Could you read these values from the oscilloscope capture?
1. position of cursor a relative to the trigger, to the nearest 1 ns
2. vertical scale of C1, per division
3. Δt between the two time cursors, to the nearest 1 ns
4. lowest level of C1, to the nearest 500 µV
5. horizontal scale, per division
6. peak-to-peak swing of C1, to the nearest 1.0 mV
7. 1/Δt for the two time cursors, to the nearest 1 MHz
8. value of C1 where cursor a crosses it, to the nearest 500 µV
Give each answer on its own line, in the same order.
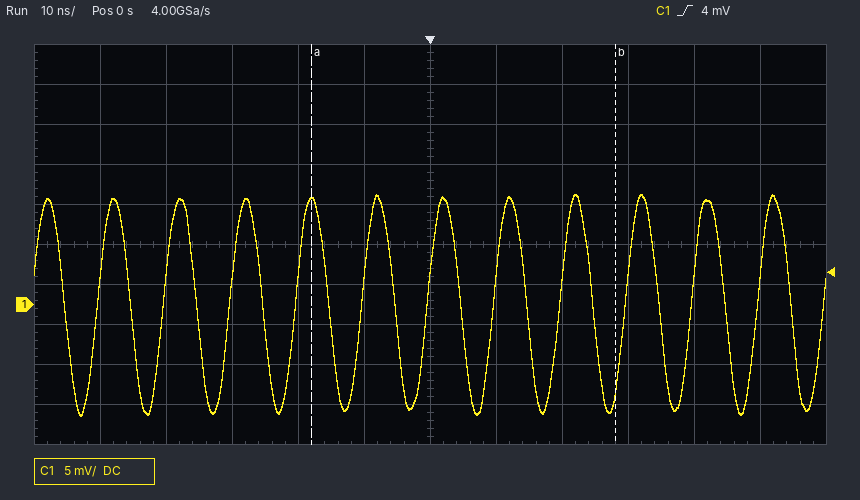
-18 ns
5 mV
46 ns
-14.0 mV
10 ns
28.0 mV
22 MHz
13.0 mV
